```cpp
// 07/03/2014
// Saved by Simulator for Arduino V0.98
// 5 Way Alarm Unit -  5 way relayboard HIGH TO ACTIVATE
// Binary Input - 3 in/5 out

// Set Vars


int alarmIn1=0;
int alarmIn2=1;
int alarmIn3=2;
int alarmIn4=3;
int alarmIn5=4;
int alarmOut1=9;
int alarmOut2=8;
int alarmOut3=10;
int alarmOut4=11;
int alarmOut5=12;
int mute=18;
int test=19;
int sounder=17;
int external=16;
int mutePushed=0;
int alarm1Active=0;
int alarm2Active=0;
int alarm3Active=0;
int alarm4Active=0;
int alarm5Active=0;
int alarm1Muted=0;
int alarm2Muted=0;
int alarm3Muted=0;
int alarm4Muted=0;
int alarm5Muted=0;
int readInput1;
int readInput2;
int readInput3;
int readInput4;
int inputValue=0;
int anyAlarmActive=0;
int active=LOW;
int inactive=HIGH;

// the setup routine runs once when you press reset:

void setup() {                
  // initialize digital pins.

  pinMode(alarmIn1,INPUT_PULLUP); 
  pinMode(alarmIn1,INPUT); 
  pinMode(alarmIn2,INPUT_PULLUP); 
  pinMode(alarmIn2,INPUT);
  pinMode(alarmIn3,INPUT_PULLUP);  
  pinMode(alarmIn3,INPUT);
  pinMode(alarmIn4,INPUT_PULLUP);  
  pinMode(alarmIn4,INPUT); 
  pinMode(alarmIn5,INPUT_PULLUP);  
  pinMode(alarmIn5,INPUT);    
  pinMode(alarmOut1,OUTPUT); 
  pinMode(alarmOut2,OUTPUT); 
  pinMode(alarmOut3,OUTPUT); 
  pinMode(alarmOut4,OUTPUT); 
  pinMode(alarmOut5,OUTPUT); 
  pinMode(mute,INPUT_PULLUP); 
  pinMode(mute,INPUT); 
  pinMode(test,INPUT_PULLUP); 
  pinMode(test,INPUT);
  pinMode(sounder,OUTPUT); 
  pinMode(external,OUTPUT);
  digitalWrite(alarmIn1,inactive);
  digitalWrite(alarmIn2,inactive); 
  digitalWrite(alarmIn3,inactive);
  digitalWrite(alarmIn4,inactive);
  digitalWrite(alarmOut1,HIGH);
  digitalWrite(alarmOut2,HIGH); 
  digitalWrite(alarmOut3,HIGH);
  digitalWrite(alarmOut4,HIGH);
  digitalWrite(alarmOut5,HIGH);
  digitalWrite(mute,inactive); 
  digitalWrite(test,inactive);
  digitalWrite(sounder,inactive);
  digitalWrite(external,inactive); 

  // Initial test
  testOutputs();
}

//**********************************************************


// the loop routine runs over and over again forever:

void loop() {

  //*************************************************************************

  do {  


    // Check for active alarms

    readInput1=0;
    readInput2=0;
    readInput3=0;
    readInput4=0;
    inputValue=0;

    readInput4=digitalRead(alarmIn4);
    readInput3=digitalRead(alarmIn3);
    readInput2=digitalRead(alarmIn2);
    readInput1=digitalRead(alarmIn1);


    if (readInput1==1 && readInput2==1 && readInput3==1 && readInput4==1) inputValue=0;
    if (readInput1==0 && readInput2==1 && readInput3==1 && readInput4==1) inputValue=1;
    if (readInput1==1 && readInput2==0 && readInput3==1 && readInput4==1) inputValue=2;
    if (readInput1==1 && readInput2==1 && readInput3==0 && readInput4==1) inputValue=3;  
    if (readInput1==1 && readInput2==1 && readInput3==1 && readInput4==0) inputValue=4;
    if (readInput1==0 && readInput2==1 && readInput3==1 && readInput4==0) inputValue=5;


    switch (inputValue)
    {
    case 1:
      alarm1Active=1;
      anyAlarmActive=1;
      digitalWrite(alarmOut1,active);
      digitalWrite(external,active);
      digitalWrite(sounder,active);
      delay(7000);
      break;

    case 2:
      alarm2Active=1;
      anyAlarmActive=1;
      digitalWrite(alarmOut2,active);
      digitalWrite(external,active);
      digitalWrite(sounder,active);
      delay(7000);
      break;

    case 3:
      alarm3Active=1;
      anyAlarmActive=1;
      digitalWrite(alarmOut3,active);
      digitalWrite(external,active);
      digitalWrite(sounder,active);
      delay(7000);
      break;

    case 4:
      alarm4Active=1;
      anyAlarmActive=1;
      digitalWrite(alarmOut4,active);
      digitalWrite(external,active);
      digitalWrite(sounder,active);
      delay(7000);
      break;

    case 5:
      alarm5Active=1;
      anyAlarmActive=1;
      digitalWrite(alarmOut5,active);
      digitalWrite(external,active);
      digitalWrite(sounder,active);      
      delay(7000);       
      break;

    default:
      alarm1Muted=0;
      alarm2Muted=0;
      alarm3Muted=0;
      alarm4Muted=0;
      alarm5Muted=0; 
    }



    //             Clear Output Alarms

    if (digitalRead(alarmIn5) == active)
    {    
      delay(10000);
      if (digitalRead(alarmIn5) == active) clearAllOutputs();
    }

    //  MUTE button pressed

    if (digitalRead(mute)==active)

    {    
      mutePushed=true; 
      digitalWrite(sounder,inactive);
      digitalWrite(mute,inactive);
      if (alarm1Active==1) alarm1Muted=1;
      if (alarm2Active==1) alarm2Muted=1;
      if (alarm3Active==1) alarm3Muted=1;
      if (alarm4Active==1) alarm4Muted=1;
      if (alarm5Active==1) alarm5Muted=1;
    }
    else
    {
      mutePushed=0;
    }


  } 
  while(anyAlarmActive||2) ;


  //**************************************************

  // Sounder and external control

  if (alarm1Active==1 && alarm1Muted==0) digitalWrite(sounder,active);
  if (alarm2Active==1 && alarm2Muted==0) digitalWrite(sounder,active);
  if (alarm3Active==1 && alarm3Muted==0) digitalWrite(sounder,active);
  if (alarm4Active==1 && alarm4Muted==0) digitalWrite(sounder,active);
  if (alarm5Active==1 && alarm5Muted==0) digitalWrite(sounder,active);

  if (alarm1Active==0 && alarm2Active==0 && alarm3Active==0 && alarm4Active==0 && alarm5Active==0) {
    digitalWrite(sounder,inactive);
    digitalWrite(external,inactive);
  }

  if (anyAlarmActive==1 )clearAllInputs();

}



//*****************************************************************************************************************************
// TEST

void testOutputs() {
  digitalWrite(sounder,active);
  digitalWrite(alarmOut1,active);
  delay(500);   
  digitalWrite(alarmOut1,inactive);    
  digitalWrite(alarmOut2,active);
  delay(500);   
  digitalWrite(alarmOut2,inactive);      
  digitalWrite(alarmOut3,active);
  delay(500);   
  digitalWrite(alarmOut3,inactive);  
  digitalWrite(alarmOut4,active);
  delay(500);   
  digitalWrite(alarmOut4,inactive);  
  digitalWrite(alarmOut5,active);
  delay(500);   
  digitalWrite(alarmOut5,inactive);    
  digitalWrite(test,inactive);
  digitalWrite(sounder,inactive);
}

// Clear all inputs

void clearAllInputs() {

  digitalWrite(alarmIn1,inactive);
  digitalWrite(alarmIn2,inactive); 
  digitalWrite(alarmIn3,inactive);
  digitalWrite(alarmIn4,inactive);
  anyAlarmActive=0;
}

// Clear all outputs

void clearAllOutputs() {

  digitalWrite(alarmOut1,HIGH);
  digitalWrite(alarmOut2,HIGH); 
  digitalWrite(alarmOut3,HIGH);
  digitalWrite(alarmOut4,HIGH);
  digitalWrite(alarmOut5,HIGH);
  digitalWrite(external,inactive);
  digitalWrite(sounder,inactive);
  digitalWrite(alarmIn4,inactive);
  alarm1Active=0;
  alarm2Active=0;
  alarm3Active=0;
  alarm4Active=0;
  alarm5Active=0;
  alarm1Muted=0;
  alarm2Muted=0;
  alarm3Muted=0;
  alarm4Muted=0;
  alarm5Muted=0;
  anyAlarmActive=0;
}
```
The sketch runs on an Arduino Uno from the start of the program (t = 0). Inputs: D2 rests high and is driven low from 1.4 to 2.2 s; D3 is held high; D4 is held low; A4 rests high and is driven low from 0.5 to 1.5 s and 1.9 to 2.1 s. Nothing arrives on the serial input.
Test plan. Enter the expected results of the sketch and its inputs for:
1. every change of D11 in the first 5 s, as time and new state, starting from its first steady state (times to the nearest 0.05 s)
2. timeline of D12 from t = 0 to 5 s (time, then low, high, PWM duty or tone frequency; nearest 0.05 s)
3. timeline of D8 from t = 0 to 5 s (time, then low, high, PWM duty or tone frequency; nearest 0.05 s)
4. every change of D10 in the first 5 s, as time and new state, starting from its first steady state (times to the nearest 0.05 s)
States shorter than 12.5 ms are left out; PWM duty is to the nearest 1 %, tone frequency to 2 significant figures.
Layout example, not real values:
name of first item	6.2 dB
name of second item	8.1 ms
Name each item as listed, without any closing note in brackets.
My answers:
every change of D11 in the first 5 s, as time and new state, starting from its first steady state	0 s high; 1.5 s low; 2 s high
timeline of D12 from t = 0 to 5 s	0 s high; 2 s low; 2.5 s high
timeline of D8 from t = 0 to 5 s	0 s high; 0.5 s low; 1 s high
every change of D10 in the first 5 s, as time and new state, starting from its first steady state	0 s high; 1 s low; 1.5 s high
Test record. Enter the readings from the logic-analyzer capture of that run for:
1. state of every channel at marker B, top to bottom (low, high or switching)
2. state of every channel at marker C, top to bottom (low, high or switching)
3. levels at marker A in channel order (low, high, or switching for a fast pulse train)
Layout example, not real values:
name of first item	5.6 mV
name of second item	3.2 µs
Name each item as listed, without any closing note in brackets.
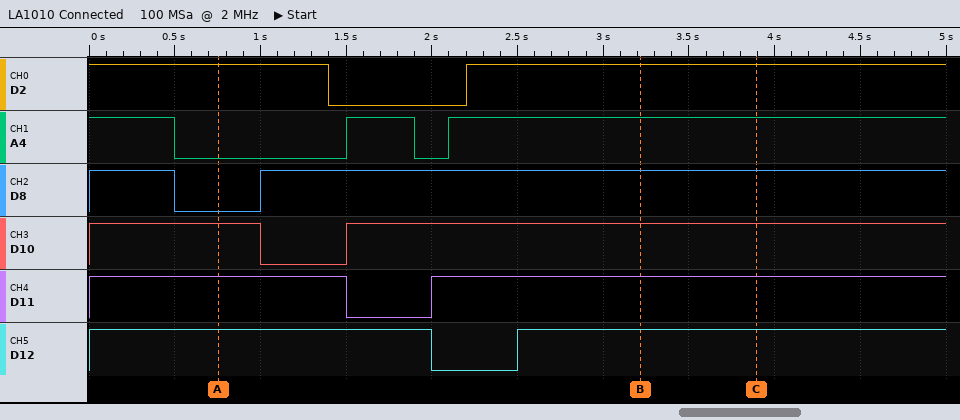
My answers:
state of every channel at marker B, top to bottom	D2 high, A4 high, D8 high, D10 high, D11 high, D12 high
state of every channel at marker C, top to bottom	D2 high, A4 high, D8 high, D10 high, D11 high, D12 high
levels at marker A in channel order	D2 high, A4 low, D8 low, D10 high, D11 high, D12 high
